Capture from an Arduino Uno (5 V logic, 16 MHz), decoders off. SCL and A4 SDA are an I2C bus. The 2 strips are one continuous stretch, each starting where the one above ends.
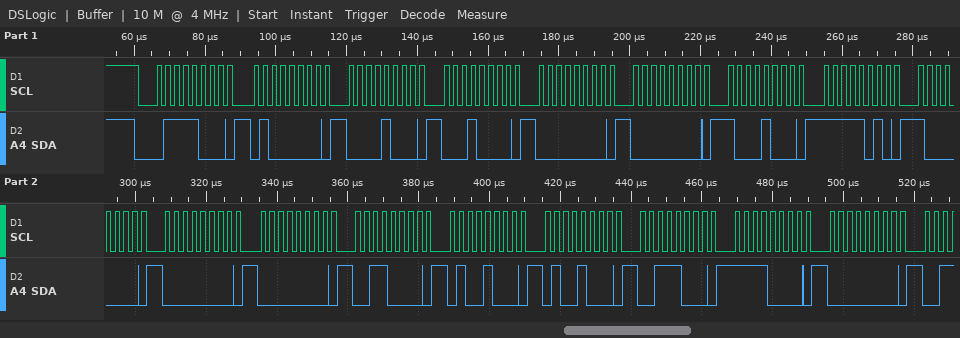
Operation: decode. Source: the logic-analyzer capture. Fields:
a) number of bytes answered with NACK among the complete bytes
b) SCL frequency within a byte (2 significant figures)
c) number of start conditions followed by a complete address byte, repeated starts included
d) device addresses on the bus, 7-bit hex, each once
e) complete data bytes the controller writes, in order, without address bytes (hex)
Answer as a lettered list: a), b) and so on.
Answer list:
a) 0
b) 400 kHz
c) 1
d) 0x3C
e) 40 08 10 00 00 88 FA 80 00 00 30 48 48 38 F0 00
